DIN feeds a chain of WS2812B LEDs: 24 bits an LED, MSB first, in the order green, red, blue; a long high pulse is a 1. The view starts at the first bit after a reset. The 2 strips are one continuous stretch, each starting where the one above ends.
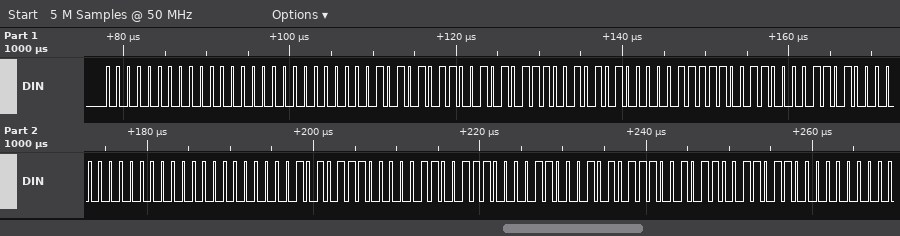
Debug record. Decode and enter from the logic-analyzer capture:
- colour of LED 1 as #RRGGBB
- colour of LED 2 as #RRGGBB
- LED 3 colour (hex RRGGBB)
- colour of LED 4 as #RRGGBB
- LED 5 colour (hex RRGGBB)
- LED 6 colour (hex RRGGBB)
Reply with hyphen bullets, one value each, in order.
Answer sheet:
- #000000
- #CA2AE5
- #F3410D
- #000000
- #0CAEE1
- #E58A9B
